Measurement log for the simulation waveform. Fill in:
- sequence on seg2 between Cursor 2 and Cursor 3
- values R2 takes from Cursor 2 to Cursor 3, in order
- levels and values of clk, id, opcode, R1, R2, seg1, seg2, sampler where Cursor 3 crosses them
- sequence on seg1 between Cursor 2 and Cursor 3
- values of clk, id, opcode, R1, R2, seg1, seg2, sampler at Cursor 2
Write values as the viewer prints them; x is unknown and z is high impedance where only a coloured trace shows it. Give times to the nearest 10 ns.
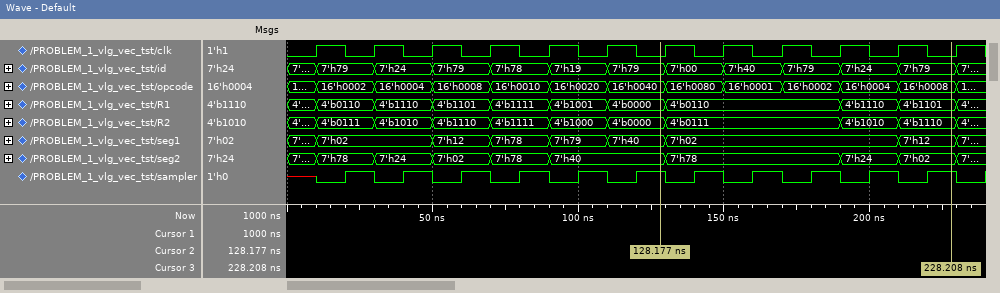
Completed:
7'h40, 7'h78, 7'h24, 7'h02
4'b0000, 4'b0111, 4'b1010, 4'b1110
clk=0, id=7'h79, opcode=16'h0008, R1=4'b1101, R2=4'b1110, seg1=7'h12, seg2=7'h02, sampler=1
7'h40, 7'h02, 7'h12
clk=0, id=7'h79, opcode=16'h0040, R1=4'b0000, R2=4'b0000, seg1=7'h40, seg2=7'h40, sampler=1
